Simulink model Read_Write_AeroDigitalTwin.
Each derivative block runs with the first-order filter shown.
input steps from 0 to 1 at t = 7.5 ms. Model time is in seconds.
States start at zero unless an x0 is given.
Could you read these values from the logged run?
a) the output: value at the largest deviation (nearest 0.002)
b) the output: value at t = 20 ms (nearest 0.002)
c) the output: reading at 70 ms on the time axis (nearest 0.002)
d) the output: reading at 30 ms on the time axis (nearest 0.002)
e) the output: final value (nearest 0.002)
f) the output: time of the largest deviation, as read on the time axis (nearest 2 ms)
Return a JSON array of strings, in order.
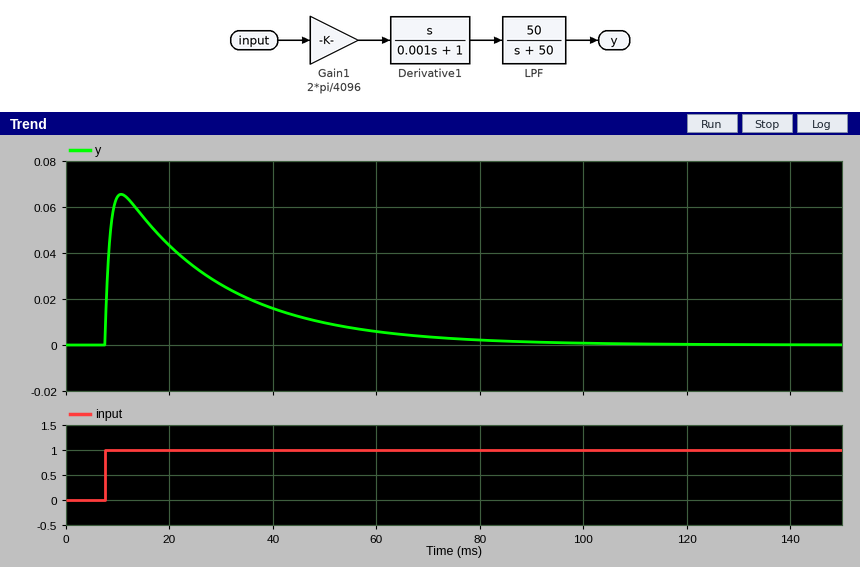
["0.066", "0.044", "0.004", "0.026", "0.000", "10 ms"]
